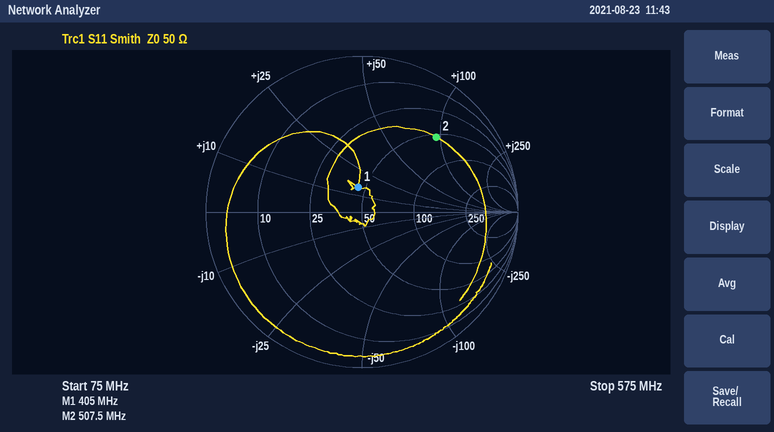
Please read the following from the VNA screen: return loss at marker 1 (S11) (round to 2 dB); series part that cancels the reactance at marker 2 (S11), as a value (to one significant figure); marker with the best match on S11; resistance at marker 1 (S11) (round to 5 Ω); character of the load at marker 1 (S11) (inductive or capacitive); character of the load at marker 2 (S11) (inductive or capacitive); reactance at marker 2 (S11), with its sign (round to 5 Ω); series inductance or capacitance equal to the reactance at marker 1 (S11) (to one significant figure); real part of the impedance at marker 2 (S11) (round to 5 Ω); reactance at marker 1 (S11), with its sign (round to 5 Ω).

16 dB
3 pF
marker 1
45 Ω
inductive
inductive
+95 Ω
6 nH
55 Ω
+15 Ω
